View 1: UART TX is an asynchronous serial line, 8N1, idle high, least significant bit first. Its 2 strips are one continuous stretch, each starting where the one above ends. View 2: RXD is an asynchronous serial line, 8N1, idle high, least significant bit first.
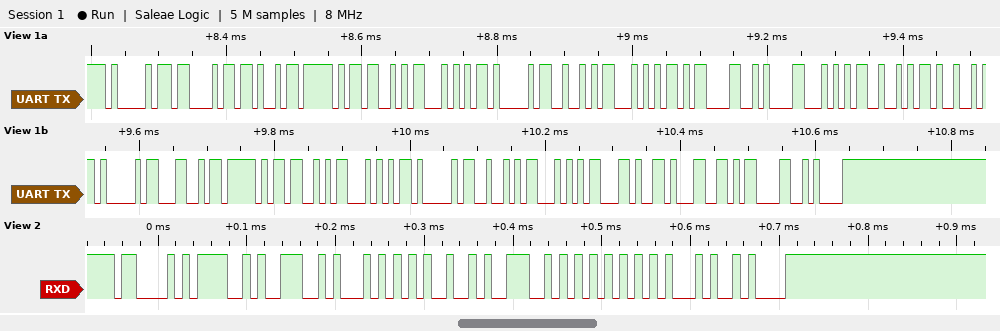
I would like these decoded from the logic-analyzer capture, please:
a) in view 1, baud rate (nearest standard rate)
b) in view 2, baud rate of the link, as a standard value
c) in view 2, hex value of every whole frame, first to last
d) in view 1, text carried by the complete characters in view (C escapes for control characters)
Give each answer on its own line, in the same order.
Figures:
115200 baud
115200 baud
43 4F 4E 54 49 4E 55 45 0A
"ACK_START\r\nTRIAL_START,1\r\n"
